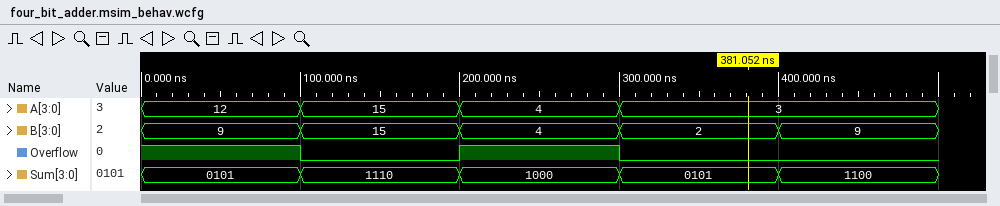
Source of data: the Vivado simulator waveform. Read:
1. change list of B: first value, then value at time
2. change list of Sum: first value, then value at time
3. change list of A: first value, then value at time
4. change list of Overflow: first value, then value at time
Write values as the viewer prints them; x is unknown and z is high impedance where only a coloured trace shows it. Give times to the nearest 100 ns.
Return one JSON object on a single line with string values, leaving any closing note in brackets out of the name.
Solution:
{"change list of B: first value, then value at time": "9, 15 at 100 ns, 4 at 200 ns, 2 at 300 ns, 9 at 400 ns", "change list of Sum: first value, then value at time": "0101, 1110 at 100 ns, 1000 at 200 ns, 0101 at 300 ns, 1100 at 400 ns", "change list of A: first value, then value at time": "12, 15 at 100 ns, 4 at 200 ns, 3 at 300 ns", "change list of Overflow: first value, then value at time": "1, 0 at 100 ns, 1 at 200 ns, 0 at 300 ns"}
